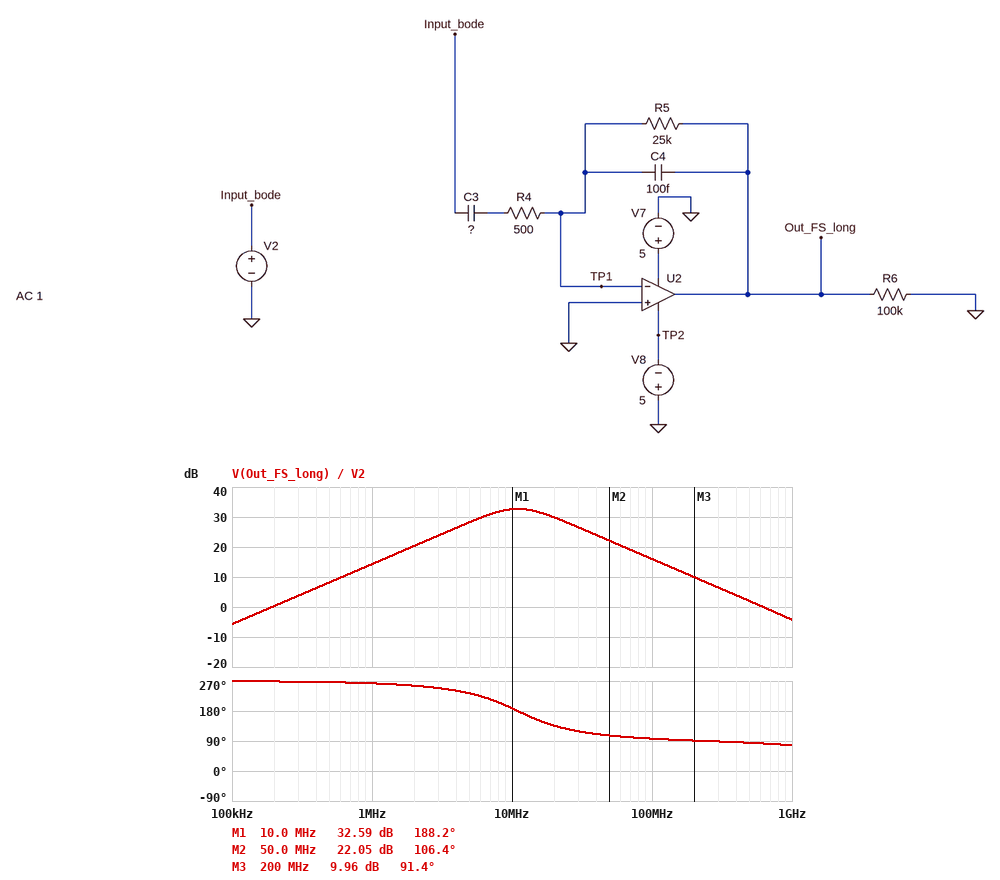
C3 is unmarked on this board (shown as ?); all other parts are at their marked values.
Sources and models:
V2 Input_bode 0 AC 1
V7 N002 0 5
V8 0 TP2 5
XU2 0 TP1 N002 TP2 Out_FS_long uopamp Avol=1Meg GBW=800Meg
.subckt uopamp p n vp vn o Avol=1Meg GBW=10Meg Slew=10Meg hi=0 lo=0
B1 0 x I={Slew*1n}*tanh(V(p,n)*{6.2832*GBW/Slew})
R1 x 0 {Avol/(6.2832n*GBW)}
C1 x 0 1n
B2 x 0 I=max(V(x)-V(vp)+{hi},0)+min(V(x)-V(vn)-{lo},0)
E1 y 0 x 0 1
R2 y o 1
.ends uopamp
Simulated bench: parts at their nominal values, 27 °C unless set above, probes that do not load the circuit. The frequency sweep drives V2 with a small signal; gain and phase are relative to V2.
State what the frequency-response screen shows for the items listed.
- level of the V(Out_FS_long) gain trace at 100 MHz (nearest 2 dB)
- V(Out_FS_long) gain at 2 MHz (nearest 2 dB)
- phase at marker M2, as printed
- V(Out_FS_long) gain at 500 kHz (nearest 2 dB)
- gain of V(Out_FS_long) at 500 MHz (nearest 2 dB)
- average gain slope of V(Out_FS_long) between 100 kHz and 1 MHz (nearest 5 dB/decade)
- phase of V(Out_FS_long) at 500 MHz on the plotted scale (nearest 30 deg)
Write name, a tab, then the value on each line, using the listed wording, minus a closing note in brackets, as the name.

level of the V(Out_FS_long) gain trace at 100 MHz	16 dB
V(Out_FS_long) gain at 2 MHz	20 dB
phase at marker M2, as printed	106.4 deg
V(Out_FS_long) gain at 500 kHz	8 dB
gain of V(Out_FS_long) at 500 MHz	2 dB
average gain slope of V(Out_FS_long) between 100 kHz and 1 MHz	20 dB/decade
phase of V(Out_FS_long) at 500 MHz on the plotted scale	90 deg
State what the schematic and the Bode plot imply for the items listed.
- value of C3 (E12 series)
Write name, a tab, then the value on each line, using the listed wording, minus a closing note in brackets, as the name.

value of C3	33 pF
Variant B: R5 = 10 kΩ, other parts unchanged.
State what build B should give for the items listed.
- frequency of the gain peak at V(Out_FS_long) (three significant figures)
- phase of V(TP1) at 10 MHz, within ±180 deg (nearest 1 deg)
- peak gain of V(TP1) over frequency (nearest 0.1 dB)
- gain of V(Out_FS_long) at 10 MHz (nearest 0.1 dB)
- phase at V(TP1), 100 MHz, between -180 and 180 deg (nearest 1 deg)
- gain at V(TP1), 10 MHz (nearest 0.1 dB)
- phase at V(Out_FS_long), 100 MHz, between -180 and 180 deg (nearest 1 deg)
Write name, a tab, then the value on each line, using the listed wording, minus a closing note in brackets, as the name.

frequency of the gain peak at V(Out_FS_long)	17.3 MHz
phase of V(TP1) at 10 MHz, within ±180 deg	121 deg
peak gain of V(TP1) over frequency	-2.3 dB
gain of V(Out_FS_long) at 10 MHz	24.1 dB
phase at V(TP1), 100 MHz, between -180 and 180 deg	17 deg
gain at V(TP1), 10 MHz	-14.0 dB
phase at V(Out_FS_long), 100 MHz, between -180 and 180 deg	107 deg
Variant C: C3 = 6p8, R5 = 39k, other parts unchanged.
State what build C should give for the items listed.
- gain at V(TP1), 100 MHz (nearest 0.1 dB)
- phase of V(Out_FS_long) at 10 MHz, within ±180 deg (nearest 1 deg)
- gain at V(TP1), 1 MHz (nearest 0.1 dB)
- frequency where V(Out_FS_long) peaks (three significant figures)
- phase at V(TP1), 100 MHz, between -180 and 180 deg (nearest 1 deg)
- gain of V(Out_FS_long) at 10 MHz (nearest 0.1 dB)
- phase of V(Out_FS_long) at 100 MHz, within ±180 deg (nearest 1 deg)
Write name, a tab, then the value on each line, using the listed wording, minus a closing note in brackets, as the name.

gain at V(TP1), 100 MHz	-1.9 dB
phase of V(Out_FS_long) at 10 MHz, within ±180 deg	-123 deg
gain at V(TP1), 1 MHz	-53.6 dB
frequency where V(Out_FS_long) peaks	19.4 MHz
phase at V(TP1), 100 MHz, between -180 and 180 deg	9 deg
gain of V(Out_FS_long) at 10 MHz	25.6 dB
phase of V(Out_FS_long) at 100 MHz, within ±180 deg	99 deg
